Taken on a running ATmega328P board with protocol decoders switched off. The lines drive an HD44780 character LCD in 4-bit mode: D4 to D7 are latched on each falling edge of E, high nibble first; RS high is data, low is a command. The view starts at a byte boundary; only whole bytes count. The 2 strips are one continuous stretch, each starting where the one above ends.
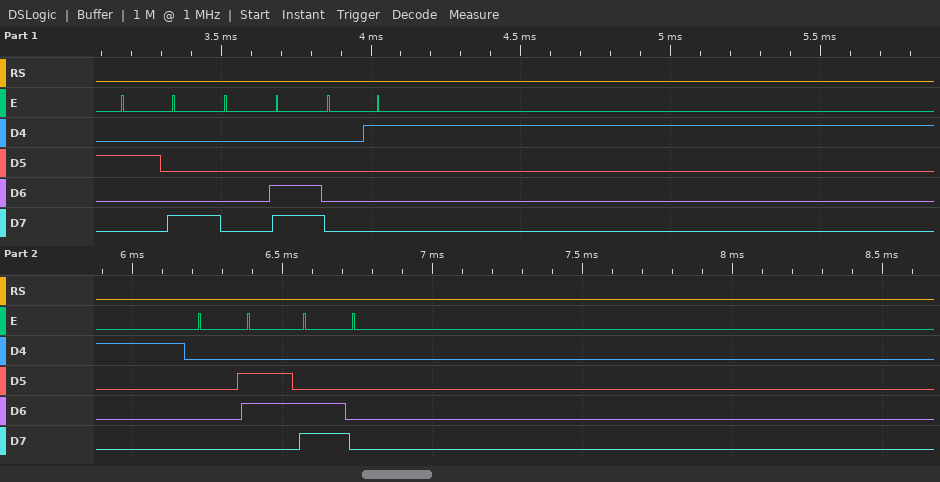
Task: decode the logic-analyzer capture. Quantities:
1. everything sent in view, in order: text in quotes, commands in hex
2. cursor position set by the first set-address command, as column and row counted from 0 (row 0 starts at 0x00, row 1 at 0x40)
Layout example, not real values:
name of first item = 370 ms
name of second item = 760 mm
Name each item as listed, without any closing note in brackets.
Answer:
everything sent in view, in order: text in quotes, commands in hex = 0x28 0x0C 0x01 0x06 0xC0
cursor position set by the first set-address command, as column and row counted from 0 = column 0, row 1
